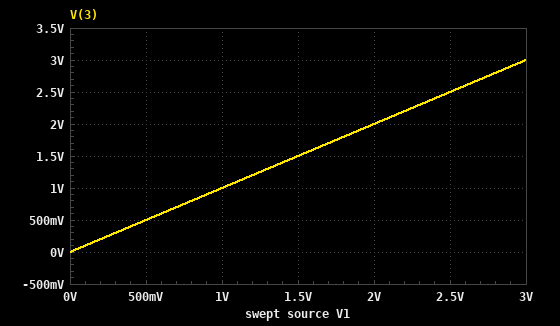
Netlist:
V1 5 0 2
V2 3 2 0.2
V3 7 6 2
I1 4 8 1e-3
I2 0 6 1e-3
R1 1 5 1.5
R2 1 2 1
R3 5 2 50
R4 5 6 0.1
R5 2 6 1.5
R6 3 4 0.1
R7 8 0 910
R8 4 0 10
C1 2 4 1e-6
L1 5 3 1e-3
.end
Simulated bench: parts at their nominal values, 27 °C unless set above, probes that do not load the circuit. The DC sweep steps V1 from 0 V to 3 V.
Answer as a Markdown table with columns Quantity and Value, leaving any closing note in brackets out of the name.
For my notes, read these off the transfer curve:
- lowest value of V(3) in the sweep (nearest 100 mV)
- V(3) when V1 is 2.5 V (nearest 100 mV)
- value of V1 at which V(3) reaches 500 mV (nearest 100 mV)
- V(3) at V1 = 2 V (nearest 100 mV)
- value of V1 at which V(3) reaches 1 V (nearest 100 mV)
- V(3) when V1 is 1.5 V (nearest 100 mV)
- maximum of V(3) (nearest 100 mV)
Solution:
| Quantity | Value |
|---|---|
| lowest value of V(3) in the sweep | 0 V |
| V(3) when V1 is 2.5 V | 2.5 V |
| value of V1 at which V(3) reaches 500 mV | 500 mV |
| V(3) at V1 = 2 V | 2.0 V |
| value of V1 at which V(3) reaches 1 V | 1.0 V |
| V(3) when V1 is 1.5 V | 1.5 V |
| maximum of V(3) | 3.0 V |
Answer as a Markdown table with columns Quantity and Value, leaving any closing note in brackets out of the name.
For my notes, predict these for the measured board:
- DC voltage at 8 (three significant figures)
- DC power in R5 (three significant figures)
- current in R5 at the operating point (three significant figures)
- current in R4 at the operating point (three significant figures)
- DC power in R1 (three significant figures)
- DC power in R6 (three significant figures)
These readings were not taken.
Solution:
| Quantity | Value |
|---|---|
| DC voltage at 8 | 910 mV |
| DC power in R5 | 23.5 mW |
| current in R5 at the operating point | 125 mA |
| current in R4 at the operating point | 124 mA |
| DC power in R1 | 9.60 mW |
| DC power in R6 | 3.96 mW |
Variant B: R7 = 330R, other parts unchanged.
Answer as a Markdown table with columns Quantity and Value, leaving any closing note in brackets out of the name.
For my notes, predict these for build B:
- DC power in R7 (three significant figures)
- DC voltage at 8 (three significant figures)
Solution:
| Quantity | Value |
|---|---|
| DC power in R7 | 330 µW |
| DC voltage at 8 | 330 mV |
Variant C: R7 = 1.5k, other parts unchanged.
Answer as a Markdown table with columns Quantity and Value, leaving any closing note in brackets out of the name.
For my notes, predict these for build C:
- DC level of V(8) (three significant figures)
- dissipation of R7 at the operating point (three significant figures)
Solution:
| Quantity | Value |
|---|---|
| DC level of V(8) | 1.50 V |
| dissipation of R7 at the operating point | 1.50 mW |
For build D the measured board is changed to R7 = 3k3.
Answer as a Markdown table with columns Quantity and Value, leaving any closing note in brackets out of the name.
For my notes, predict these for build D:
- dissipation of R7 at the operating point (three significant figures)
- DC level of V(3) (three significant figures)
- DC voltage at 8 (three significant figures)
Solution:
| Quantity | Value |
|---|---|
| dissipation of R7 at the operating point | 3.30 mW |
| DC level of V(3) | 2.00 V |
| DC voltage at 8 | 3.30 V |
